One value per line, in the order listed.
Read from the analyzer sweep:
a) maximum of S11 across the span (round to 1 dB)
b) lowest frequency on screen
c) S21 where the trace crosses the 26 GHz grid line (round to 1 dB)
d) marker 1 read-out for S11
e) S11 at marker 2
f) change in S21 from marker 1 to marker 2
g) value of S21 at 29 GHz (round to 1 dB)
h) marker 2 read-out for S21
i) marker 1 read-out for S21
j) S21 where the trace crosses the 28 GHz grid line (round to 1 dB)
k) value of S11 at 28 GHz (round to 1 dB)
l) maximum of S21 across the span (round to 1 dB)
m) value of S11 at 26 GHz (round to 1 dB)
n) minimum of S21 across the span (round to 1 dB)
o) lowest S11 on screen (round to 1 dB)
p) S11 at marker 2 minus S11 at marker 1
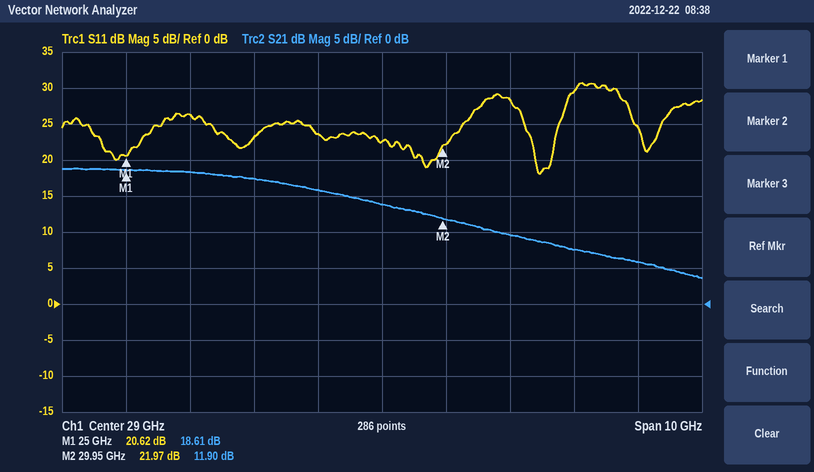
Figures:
31 dB
24 GHz
18 dB
20.62 dB
21.97 dB
-6.71 dB
14 dB
11.90 dB
18.61 dB
16 dB
24 dB
19 dB
26 dB
4 dB
18 dB
1.35 dB
